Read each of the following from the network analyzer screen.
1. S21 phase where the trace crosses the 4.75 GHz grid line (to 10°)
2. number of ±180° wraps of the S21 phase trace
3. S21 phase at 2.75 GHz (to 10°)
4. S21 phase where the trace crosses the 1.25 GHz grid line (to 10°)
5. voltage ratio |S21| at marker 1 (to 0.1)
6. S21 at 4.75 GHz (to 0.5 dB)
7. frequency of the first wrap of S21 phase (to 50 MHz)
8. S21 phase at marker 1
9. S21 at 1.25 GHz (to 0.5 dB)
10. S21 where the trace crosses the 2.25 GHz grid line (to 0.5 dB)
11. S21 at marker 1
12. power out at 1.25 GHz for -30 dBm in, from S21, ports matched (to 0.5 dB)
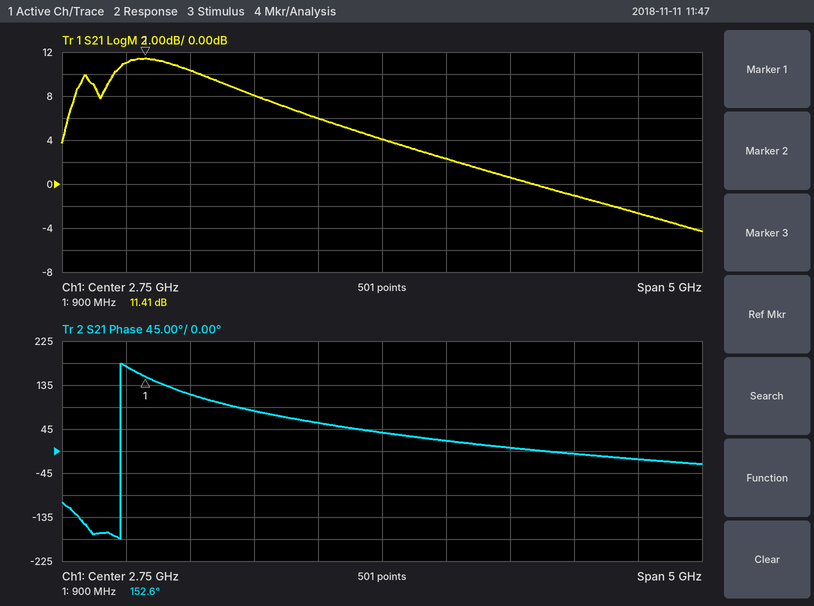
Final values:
-20°
1
40°
120°
3.7
-2.5 dB
700 MHz
152.6°
10.5 dB
6.0 dB
11.41 dB
-19.5 dBm
